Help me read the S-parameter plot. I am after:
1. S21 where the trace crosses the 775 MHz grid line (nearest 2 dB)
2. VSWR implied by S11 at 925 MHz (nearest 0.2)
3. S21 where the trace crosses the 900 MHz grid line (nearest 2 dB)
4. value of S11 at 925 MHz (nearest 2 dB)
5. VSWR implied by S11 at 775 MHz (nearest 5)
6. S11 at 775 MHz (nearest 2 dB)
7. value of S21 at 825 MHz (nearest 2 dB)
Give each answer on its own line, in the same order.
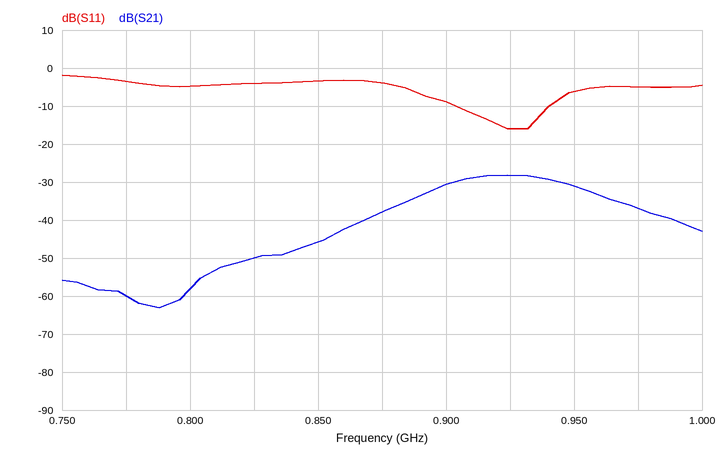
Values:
-60 dB
1.4
-30 dB
-16 dB
5
-4 dB
-50 dB
